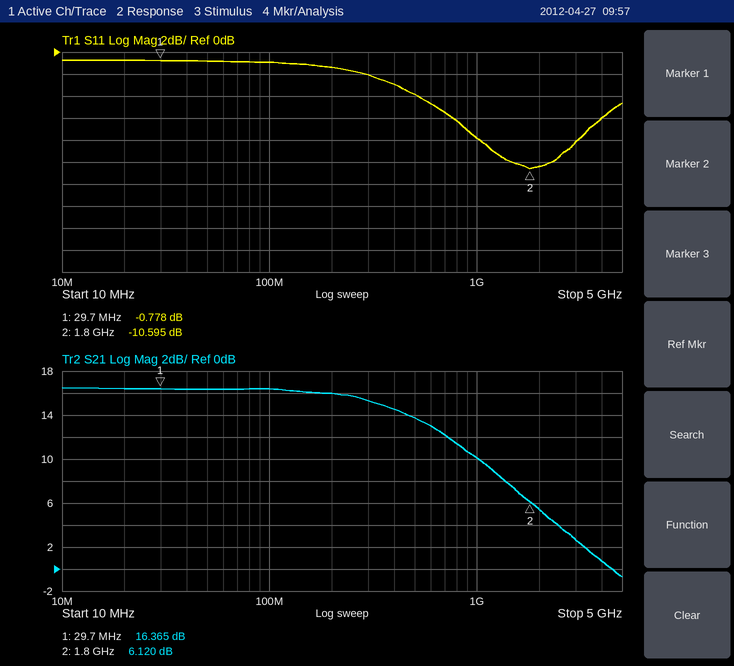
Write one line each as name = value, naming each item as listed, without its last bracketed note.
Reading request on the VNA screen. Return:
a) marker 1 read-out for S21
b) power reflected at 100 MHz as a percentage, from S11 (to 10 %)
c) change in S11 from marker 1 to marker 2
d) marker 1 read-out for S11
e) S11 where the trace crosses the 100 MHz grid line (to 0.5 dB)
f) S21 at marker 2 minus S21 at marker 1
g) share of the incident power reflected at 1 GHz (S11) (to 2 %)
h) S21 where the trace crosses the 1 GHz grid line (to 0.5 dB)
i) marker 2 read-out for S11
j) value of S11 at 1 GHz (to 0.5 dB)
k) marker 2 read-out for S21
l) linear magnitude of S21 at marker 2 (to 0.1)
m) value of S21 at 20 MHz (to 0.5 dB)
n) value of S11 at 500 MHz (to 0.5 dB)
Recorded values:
marker 1 read-out for S21 = 16.365 dB
power reflected at 100 MHz as a percentage, from S11 = 80 %
change in S11 from marker 1 to marker 2 = -9.817 dB
marker 1 read-out for S11 = -0.778 dB
S11 where the trace crosses the 100 MHz grid line = -1.0 dB
S21 at marker 2 minus S21 at marker 1 = -10.245 dB
share of the incident power reflected at 1 GHz (S11) = 16 %
S21 where the trace crosses the 1 GHz grid line = 10.0 dB
marker 2 read-out for S11 = -10.595 dB
value of S11 at 1 GHz = -8.0 dB
marker 2 read-out for S21 = 6.120 dB
linear magnitude of S21 at marker 2 = 2.0
value of S21 at 20 MHz = 16.5 dB
value of S11 at 500 MHz = -4.0 dB
